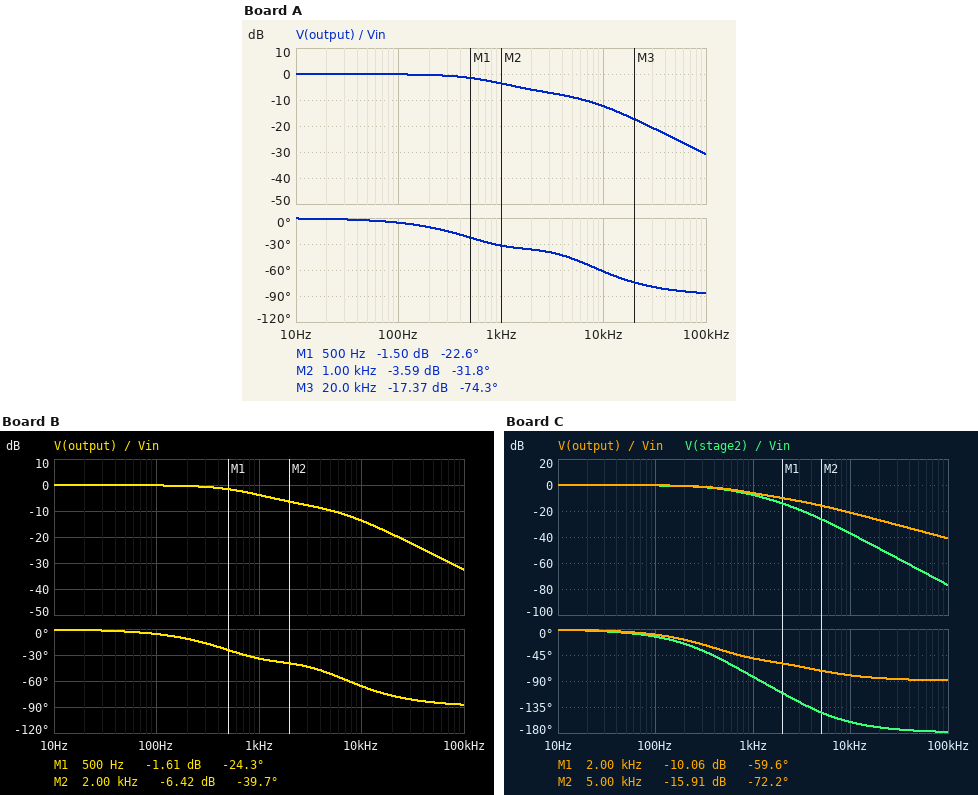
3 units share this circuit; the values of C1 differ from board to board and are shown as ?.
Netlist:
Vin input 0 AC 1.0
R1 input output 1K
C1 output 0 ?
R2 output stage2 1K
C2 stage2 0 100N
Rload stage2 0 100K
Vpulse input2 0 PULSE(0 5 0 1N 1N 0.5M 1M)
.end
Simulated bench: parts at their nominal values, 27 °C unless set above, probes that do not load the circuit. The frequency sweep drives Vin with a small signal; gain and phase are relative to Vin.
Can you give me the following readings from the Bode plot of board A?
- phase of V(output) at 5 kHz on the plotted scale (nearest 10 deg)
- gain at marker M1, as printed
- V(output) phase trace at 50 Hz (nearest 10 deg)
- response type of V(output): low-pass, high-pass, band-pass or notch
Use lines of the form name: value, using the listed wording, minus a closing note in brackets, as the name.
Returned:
phase of V(output) at 5 kHz on the plotted scale: -50 deg
gain at marker M1, as printed: -1.50 dB
V(output) phase trace at 50 Hz: 0 deg
response type of V(output): low-pass, high-pass, band-pass or notch: low-pass
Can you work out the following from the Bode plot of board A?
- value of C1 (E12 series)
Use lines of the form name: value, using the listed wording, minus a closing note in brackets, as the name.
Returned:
value of C1: 56 nF
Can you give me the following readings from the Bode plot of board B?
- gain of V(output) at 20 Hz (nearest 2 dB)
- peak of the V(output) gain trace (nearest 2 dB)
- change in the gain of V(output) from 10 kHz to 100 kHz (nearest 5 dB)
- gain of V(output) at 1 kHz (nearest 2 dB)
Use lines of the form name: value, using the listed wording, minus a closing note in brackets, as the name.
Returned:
gain of V(output) at 20 Hz: 0 dB
peak of the V(output) gain trace: 0 dB
change in the gain of V(output) from 10 kHz to 100 kHz: -20 dB
gain of V(output) at 1 kHz: -4 dB
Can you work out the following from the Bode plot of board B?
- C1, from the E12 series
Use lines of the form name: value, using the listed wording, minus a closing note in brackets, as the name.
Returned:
C1, from the E12 series: 68 nF
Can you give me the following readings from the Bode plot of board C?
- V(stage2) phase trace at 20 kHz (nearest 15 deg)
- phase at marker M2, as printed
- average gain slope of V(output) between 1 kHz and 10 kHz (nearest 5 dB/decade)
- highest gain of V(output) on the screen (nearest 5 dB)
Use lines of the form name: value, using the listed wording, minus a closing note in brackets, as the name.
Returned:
V(stage2) phase trace at 20 kHz: -165 deg
phase at marker M2, as printed: -72.2 deg
average gain slope of V(output) between 1 kHz and 10 kHz: -15 dB/decade
highest gain of V(output) on the screen: 0 dB
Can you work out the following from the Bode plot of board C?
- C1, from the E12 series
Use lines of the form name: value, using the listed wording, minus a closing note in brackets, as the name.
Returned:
C1, from the E12 series: 180 nF
